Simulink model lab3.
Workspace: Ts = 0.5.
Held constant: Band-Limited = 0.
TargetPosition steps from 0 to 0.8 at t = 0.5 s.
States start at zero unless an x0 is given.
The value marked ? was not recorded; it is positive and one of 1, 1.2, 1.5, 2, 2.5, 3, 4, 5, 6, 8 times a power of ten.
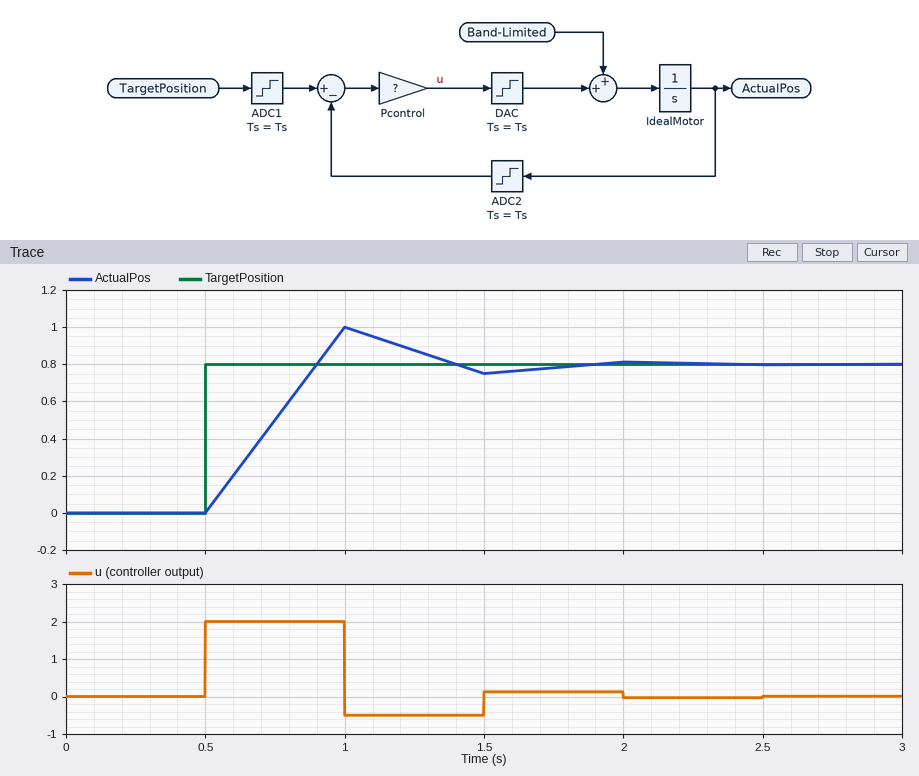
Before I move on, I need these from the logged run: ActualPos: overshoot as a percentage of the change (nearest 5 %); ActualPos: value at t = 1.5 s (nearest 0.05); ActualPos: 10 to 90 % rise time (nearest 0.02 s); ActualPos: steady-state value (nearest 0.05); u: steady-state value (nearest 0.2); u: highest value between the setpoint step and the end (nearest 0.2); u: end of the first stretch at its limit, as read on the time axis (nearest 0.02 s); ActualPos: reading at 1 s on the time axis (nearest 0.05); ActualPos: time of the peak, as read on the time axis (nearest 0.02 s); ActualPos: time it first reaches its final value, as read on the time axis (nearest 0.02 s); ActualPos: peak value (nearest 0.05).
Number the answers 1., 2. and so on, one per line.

1. 25 %
2. 0.75
3. 0.32 s
4. 0.80
5. 0.0
6. 2.0
7. 1.00 s
8. 1.00
9. 1.00 s
10. 0.90 s
11. 1.00
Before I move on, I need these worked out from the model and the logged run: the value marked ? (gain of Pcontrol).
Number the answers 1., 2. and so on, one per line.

1. 2.5
